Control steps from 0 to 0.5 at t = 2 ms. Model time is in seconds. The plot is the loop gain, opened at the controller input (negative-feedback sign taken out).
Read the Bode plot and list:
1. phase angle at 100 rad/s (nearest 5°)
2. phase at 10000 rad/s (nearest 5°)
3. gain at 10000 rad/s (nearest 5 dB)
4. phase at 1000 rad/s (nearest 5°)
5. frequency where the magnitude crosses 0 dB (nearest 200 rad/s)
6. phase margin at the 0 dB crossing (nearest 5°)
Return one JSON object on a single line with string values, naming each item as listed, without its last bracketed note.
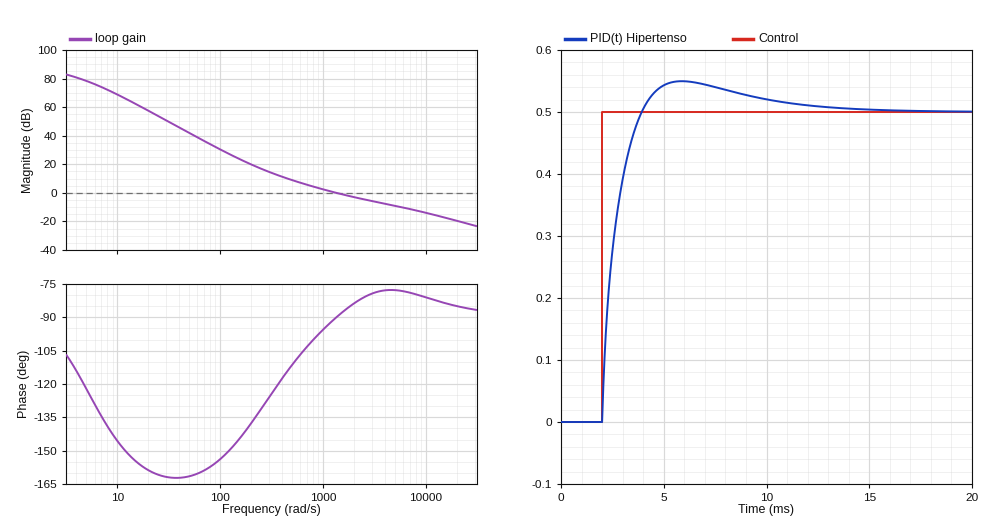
{"phase angle at 100 rad/s": "-155°", "phase at 10000 rad/s": "-80°", "gain at 10000 rad/s": "-15 dB", "phase at 1000 rad/s": "-95°", "frequency where the magnitude crosses 0 dB": "1400 rad/s", "phase margin at the 0 dB crossing": "90°"}
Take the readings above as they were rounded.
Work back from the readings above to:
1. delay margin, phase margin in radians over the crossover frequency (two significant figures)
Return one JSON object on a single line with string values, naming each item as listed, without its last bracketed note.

{"delay margin, phase margin in radians over the crossover frequency": "0.0011 s"}
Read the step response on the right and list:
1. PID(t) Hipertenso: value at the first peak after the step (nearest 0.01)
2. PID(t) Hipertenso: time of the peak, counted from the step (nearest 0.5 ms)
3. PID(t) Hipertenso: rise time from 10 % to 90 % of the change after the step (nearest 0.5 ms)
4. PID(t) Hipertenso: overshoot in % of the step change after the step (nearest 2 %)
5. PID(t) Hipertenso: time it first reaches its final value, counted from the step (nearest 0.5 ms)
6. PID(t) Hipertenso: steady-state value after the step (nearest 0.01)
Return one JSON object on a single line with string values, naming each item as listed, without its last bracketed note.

{"PID(t) Hipertenso: value at the first peak after the step": "0.55", "PID(t) Hipertenso: time of the peak, counted from the step": "4.0 ms", "PID(t) Hipertenso: rise time from 10 % to 90 % of the change after the step": "1.5 ms", "PID(t) Hipertenso: overshoot in % of the step change after the step": "10 %", "PID(t) Hipertenso: time it first reaches its final value, counted from the step": "2.0 ms", "PID(t) Hipertenso: steady-state value after the step": "0.50"}
